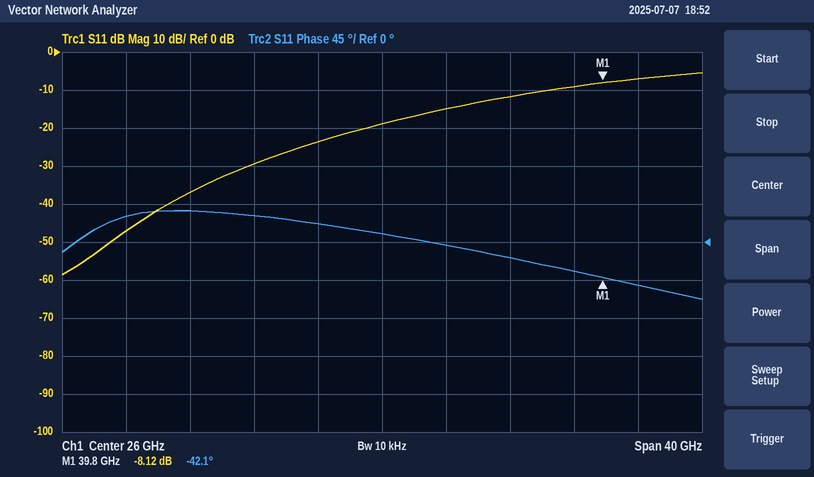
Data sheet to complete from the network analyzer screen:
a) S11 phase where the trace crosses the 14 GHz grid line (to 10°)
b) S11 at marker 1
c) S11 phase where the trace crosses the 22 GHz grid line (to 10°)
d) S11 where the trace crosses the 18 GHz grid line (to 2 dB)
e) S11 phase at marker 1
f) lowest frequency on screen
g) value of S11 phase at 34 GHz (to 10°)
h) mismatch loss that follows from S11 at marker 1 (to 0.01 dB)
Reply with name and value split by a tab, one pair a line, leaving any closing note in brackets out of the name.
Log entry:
S11 phase where the trace crosses the 14 GHz grid line	40°
S11 at marker 1	-8.12 dB
S11 phase where the trace crosses the 22 GHz grid line	20°
S11 where the trace crosses the 18 GHz grid line	-30 dB
S11 phase at marker 1	-42.1°
lowest frequency on screen	6 GHz
value of S11 phase at 34 GHz	-20°
mismatch loss that follows from S11 at marker 1	0.73 dB
